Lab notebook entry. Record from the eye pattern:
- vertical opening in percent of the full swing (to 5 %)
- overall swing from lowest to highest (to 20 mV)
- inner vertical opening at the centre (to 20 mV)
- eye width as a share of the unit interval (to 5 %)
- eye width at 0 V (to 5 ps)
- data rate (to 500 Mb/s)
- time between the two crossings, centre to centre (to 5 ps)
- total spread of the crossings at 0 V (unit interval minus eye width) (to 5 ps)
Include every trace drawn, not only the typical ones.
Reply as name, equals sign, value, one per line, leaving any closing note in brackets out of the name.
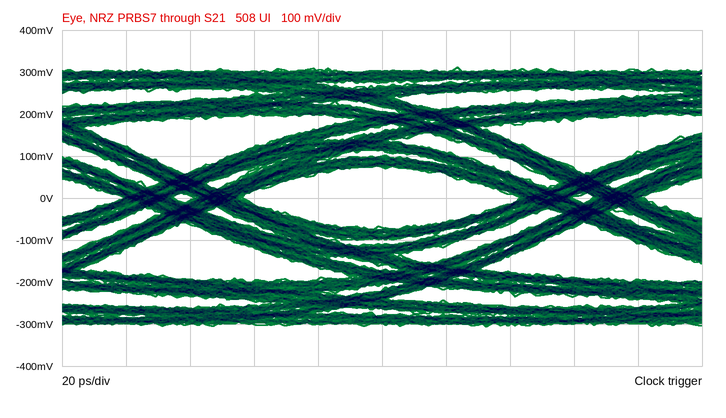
vertical opening in percent of the full swing = 25 %
overall swing from lowest to highest = 620 mV
inner vertical opening at the centre = 140 mV
eye width as a share of the unit interval = 70 %
eye width at 0 V = 85 ps
data rate = 8.0 Gb/s
time between the two crossings, centre to centre = 125 ps
total spread of the crossings at 0 V (unit interval minus eye width) = 40 ps
